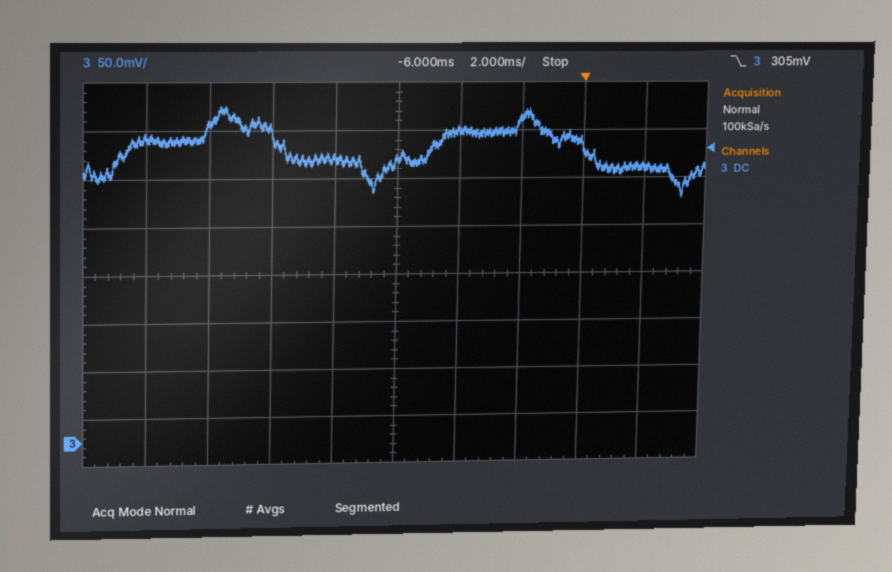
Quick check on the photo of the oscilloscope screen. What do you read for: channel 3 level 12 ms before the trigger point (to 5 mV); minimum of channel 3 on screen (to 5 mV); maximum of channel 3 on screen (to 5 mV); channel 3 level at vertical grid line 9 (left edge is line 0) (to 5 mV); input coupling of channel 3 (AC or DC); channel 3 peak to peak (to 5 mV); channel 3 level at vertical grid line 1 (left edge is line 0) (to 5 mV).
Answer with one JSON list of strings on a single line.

["330 mV", "255 mV", "350 mV", "285 mV", "DC", "95 mV", "315 mV"]
